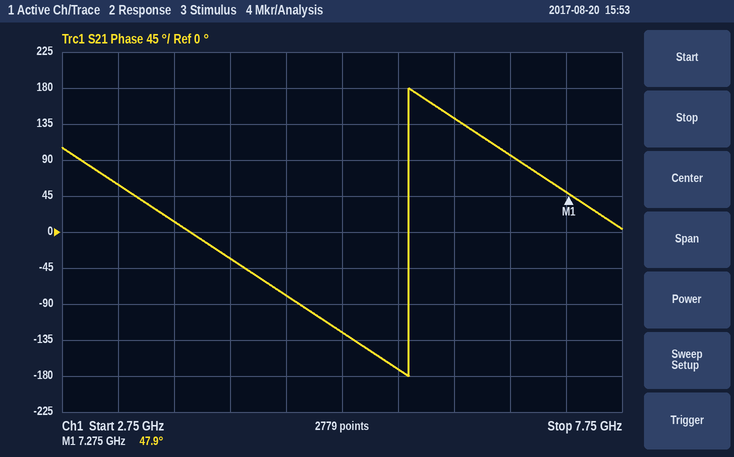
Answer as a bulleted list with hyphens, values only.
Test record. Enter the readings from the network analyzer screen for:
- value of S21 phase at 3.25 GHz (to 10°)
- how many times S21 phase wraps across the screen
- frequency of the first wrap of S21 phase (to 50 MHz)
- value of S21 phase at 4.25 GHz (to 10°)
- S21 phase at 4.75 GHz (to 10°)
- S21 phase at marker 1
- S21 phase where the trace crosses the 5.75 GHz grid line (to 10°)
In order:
- 60°
- 1
- 5.85 GHz
- -30°
- -80°
- 47.9°
- -170°
